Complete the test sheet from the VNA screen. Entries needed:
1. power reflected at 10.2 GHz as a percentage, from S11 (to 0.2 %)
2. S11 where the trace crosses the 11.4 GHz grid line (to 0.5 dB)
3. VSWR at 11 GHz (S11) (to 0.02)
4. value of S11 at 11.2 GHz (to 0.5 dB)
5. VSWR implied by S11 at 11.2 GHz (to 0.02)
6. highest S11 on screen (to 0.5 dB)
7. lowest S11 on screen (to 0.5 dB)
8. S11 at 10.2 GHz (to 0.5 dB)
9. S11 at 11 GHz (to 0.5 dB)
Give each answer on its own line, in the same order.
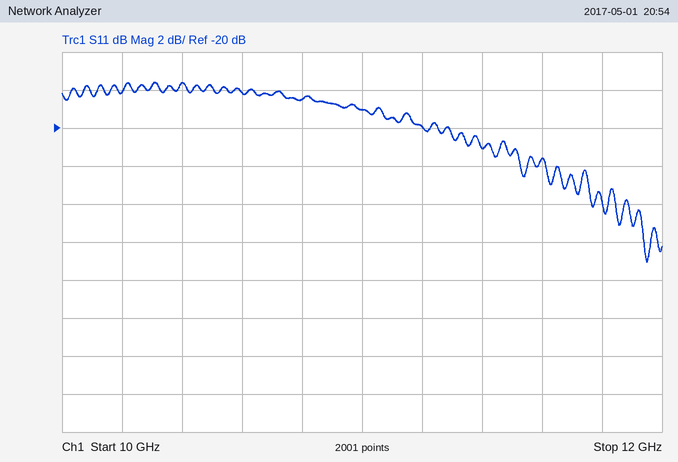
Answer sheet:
1.6 %
-21.0 dB
1.26
-20.0 dB
1.22
-17.5 dB
-27.0 dB
-18.0 dB
-19.0 dB
